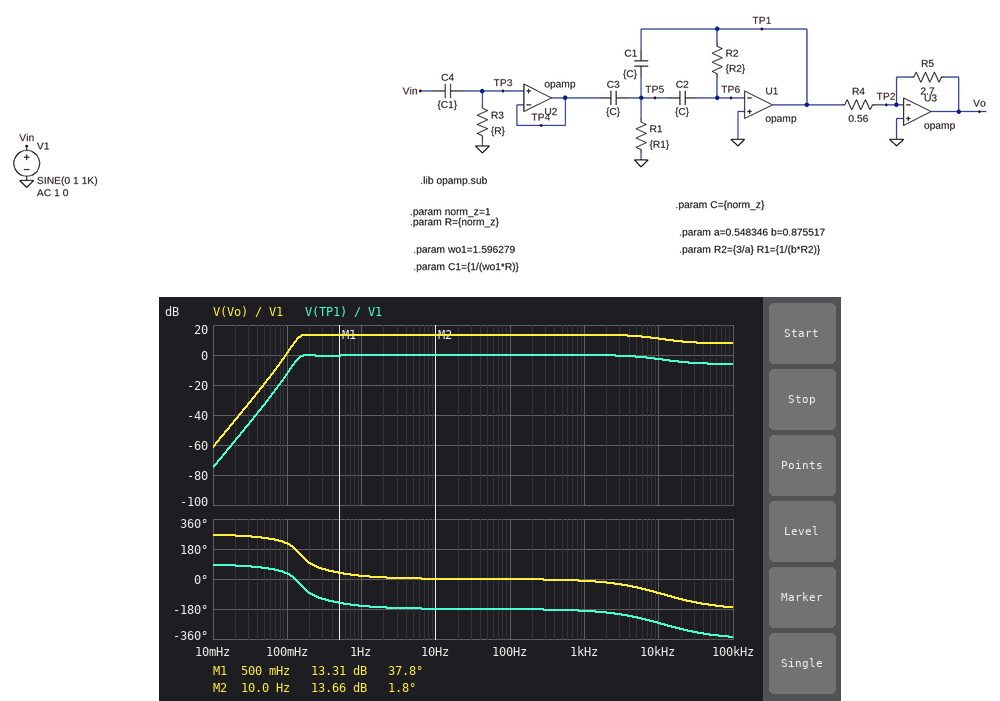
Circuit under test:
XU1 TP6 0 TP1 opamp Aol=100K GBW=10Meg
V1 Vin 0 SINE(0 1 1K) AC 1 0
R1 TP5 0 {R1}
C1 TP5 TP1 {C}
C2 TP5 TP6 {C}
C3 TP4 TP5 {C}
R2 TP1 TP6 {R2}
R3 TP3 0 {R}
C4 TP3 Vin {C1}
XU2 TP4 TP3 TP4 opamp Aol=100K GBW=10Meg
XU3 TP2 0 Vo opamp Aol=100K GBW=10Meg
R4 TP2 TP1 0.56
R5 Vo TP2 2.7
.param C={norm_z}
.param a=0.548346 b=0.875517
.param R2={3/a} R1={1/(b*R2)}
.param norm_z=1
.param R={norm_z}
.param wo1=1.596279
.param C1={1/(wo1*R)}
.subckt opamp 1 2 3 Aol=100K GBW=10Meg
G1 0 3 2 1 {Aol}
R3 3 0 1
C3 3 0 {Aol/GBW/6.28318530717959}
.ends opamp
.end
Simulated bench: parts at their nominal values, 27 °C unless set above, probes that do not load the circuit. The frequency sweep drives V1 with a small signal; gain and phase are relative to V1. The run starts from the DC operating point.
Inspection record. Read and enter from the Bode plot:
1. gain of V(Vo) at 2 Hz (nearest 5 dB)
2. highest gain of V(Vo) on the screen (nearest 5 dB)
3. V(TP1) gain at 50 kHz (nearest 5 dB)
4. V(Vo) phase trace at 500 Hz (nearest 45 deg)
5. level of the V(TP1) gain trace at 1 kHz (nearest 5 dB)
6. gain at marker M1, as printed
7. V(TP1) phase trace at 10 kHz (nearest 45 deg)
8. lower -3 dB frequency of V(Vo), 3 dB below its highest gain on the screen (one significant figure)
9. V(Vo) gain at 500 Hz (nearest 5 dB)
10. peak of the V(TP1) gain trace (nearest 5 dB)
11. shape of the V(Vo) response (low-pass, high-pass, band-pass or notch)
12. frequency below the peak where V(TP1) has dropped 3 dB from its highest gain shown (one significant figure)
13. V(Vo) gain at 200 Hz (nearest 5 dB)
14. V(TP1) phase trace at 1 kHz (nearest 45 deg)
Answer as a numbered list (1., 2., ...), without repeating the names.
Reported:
1. 15 dB
2. 15 dB
3. -5 dB
4. 0 deg
5. 0 dB
6. 13.31 dB
7. -270 deg
8. 100 mHz
9. 15 dB
10. 0 dB
11. high-pass
12. 100 mHz
13. 15 dB
14. -180 deg
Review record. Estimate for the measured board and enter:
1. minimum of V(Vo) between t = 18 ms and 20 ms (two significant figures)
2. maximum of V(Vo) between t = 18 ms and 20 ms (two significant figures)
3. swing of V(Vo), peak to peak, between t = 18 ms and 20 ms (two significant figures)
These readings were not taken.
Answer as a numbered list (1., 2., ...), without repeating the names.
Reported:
1. -4.8 V
2. 4.8 V
3. 9.6 V
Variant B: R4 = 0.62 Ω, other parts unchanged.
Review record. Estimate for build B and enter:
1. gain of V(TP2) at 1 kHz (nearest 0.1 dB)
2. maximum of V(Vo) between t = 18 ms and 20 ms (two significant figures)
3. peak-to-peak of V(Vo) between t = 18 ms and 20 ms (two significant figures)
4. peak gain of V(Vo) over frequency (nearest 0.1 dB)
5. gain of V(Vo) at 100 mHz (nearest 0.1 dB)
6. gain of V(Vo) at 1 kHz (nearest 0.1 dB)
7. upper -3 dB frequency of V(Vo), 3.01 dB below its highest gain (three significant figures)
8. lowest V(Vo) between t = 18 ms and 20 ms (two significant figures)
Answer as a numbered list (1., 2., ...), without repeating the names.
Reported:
1. -67.2 dB
2. 4.3 V
3. 8.7 V
4. 12.8 dB
5. 0.5 dB
6. 12.7 dB
7. 11.2 kHz
8. -4.3 V
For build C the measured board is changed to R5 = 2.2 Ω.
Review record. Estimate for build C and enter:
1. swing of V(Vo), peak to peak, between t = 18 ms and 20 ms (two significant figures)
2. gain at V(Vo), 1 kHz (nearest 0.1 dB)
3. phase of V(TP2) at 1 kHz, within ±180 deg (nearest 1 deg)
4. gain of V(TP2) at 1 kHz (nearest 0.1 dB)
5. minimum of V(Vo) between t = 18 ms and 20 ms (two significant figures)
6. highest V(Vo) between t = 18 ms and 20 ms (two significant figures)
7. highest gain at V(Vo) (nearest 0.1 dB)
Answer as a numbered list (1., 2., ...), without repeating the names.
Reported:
1. 7.8 V
2. 11.8 dB
3. -109 deg
4. -68.1 dB
5. -3.9 V
6. 3.9 V
7. 11.9 dB
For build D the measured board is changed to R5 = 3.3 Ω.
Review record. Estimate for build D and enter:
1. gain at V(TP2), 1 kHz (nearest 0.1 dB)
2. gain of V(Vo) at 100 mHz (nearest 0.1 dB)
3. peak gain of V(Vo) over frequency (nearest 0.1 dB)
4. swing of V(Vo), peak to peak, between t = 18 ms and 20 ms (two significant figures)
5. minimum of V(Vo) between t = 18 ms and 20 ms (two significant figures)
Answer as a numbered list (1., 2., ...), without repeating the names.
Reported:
1. -64.6 dB
2. 3.2 dB
3. 15.4 dB
4. 12 V
5. -5.9 V
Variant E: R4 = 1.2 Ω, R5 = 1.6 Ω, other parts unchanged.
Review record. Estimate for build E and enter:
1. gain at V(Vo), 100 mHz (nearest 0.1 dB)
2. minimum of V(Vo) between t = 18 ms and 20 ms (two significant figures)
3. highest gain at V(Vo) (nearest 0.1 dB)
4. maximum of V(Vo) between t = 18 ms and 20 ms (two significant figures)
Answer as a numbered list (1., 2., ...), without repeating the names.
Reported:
1. -9.7 dB
2. -1.3 V
3. 2.5 dB
4. 1.3 V
